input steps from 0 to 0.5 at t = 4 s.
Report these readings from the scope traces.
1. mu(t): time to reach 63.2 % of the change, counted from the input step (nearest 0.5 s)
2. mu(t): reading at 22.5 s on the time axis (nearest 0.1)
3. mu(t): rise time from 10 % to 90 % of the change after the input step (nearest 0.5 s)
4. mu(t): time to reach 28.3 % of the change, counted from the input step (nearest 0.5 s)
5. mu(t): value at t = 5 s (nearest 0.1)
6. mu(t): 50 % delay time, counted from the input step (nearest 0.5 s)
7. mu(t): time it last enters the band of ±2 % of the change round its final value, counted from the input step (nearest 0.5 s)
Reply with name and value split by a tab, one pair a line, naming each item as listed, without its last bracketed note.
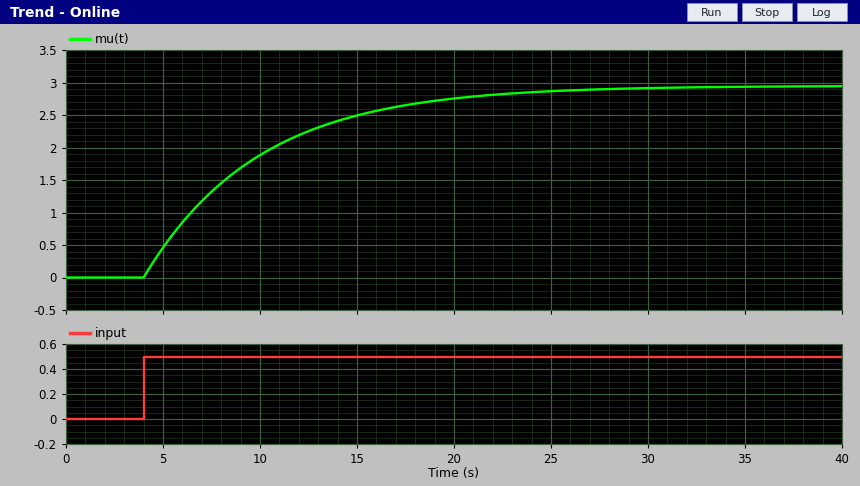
mu(t): time to reach 63.2 % of the change, counted from the input step	6.0 s
mu(t): reading at 22.5 s on the time axis	2.8
mu(t): rise time from 10 % to 90 % of the change after the input step	13.0 s
mu(t): time to reach 28.3 % of the change, counted from the input step	2.0 s
mu(t): value at t = 5 s	0.5
mu(t): 50 % delay time, counted from the input step	4.0 s
mu(t): time it last enters the band of ±2 % of the change round its final value, counted from the input step	23.0 s
